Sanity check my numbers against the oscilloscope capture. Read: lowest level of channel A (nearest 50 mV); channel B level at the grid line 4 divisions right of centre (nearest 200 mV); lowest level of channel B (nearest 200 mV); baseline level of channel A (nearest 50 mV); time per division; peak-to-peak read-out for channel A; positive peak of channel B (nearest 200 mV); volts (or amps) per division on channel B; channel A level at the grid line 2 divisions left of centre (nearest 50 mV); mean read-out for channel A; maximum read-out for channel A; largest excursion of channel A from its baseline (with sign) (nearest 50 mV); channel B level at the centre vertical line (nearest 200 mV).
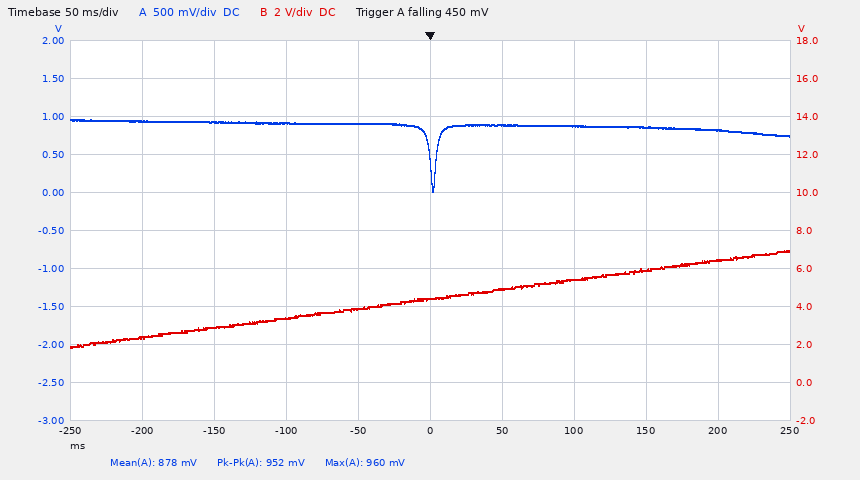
0 mV
6.4 V
1.8 V
900 mV
50 ms
952 mV
7.0 V
2 V
900 mV
878 mV
960 mV
-900 mV
4.4 V
